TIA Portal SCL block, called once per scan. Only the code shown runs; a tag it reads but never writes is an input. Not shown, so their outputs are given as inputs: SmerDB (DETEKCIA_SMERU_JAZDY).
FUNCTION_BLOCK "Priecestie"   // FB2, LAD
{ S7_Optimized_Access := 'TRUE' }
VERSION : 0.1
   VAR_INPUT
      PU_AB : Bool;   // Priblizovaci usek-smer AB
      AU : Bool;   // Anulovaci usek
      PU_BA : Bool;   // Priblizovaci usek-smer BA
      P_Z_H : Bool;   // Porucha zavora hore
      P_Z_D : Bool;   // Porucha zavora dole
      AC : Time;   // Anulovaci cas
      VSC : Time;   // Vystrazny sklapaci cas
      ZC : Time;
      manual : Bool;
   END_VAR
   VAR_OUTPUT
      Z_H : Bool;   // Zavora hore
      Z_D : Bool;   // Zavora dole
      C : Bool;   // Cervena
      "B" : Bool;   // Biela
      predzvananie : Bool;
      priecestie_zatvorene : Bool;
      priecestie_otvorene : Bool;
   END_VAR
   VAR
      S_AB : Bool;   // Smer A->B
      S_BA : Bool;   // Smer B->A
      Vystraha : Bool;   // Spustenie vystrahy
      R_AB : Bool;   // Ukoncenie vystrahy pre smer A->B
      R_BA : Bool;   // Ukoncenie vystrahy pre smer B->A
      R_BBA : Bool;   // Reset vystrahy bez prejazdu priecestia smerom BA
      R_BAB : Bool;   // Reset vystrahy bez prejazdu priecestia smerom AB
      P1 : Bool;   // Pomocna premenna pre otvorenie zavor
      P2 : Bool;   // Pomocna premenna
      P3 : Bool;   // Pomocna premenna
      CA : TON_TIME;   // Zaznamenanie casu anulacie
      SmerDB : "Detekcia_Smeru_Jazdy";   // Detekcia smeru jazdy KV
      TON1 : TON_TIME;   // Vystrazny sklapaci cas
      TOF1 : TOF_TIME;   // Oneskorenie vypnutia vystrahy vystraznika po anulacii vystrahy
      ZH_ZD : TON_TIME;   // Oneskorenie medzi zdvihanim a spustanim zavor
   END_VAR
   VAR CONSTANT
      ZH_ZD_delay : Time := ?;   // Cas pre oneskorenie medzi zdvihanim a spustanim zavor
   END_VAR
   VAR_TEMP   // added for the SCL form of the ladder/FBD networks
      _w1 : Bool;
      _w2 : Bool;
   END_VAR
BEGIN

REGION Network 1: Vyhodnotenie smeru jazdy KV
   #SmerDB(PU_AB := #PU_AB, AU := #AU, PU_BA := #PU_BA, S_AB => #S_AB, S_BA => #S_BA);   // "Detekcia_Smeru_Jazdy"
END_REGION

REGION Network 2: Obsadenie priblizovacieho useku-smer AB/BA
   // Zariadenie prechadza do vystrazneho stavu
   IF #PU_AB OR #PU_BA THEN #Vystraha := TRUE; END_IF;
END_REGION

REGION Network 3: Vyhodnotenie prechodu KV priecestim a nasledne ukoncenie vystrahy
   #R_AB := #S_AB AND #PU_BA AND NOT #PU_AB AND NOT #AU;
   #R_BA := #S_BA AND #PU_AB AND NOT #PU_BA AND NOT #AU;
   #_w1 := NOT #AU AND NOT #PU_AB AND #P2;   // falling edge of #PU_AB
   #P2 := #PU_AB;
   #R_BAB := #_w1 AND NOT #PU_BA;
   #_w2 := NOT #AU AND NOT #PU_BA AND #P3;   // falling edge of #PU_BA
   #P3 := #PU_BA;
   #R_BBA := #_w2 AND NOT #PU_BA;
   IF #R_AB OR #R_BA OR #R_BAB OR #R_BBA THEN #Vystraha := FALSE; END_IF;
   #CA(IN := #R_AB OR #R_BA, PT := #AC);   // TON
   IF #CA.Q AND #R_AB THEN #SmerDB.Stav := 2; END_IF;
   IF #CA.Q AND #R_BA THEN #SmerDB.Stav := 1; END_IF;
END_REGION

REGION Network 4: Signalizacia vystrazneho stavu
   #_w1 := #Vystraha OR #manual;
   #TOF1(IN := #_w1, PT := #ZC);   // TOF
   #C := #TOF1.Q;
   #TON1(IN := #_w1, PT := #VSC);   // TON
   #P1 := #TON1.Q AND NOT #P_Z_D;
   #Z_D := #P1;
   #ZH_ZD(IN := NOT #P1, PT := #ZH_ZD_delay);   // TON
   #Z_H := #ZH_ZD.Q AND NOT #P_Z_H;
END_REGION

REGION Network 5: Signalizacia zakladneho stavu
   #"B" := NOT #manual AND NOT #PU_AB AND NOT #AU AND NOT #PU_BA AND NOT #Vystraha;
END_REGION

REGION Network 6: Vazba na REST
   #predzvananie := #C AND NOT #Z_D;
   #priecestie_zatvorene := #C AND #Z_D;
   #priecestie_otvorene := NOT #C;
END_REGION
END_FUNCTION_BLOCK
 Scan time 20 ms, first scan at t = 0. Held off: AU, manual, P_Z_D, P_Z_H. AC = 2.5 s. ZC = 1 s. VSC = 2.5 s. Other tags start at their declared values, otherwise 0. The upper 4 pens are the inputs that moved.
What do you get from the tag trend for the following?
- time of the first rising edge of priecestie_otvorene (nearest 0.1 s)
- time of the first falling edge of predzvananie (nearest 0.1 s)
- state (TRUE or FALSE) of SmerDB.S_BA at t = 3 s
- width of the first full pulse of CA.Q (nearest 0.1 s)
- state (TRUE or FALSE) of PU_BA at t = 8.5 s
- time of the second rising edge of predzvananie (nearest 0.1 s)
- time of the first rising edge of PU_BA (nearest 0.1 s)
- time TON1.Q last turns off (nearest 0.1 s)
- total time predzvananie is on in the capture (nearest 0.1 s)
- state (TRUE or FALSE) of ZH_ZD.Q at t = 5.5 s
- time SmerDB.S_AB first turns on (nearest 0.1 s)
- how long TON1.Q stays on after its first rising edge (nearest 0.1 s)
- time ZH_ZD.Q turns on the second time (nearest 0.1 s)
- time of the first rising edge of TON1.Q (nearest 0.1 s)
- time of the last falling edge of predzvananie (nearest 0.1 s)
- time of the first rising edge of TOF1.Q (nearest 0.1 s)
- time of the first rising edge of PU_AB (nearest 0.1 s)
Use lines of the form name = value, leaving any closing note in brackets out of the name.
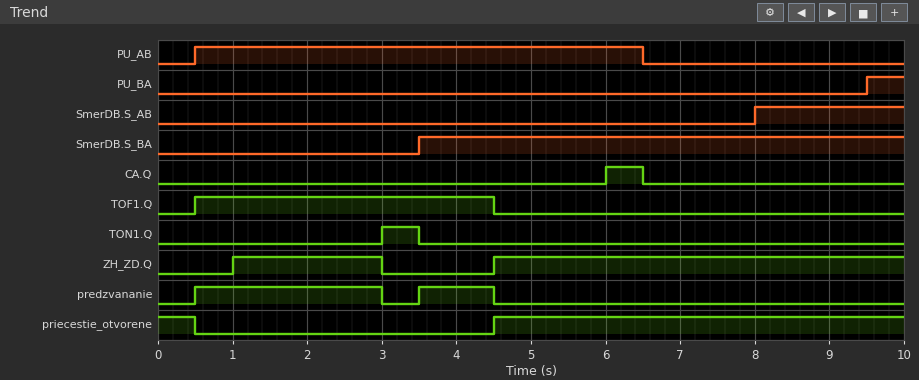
time of the first rising edge of priecestie_otvorene = 4.5 s
time of the first falling edge of predzvananie = 3.0 s
state (TRUE or FALSE) of SmerDB.S_BA at t = 3 s = FALSE
width of the first full pulse of CA.Q = 0.5 s
state (TRUE or FALSE) of PU_BA at t = 8.5 s = FALSE
time of the second rising edge of predzvananie = 3.5 s
time of the first rising edge of PU_BA = 9.5 s
time TON1.Q last turns off = 3.5 s
total time predzvananie is on in the capture = 3.5 s
state (TRUE or FALSE) of ZH_ZD.Q at t = 5.5 s = TRUE
time SmerDB.S_AB first turns on = 8.0 s
how long TON1.Q stays on after its first rising edge = 0.5 s
time ZH_ZD.Q turns on the second time = 4.5 s
time of the first rising edge of TON1.Q = 3.0 s
time of the last falling edge of predzvananie = 4.5 s
time of the first rising edge of TOF1.Q = 0.5 s
time of the first rising edge of PU_AB = 0.5 s
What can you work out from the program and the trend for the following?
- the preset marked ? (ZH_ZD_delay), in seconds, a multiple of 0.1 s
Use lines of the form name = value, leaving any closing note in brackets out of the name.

the preset marked ? (ZH_ZD_delay), in seconds, a multiple of 0.1 s = 1.0 s
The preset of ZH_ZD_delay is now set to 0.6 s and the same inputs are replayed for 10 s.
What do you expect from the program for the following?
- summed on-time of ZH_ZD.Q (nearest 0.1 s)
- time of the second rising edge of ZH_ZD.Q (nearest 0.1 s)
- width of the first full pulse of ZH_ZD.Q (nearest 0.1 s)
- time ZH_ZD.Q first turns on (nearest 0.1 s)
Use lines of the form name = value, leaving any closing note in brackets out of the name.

summed on-time of ZH_ZD.Q = 8.3 s
time of the second rising edge of ZH_ZD.Q = 4.1 s
width of the first full pulse of ZH_ZD.Q = 2.4 s
time ZH_ZD.Q first turns on = 0.6 s
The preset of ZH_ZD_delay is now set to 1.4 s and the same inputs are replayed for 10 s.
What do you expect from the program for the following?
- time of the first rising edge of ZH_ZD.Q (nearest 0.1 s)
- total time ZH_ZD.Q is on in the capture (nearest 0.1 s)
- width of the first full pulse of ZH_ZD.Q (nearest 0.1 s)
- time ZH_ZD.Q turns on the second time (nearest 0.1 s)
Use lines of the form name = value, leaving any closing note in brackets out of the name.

time of the first rising edge of ZH_ZD.Q = 1.4 s
total time ZH_ZD.Q is on in the capture = 6.7 s
width of the first full pulse of ZH_ZD.Q = 1.6 s
time ZH_ZD.Q turns on the second time = 4.9 s
